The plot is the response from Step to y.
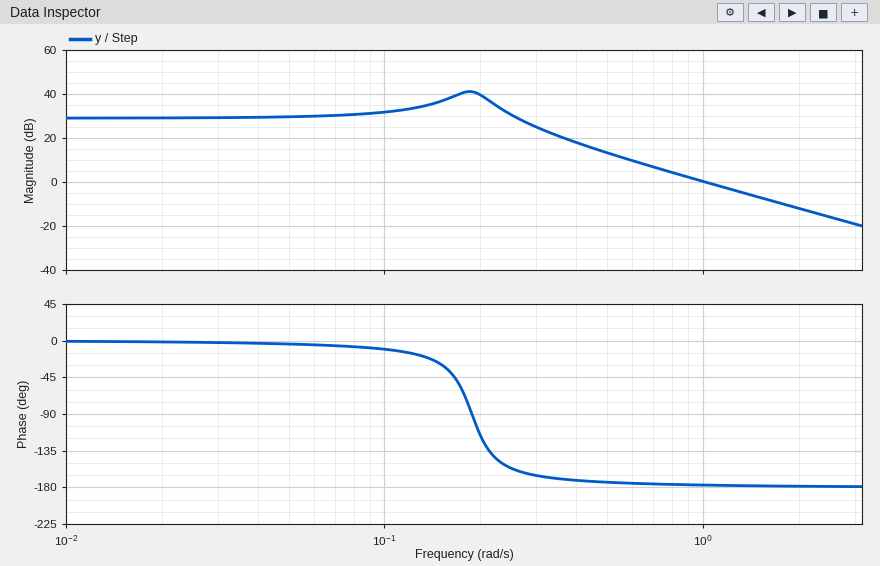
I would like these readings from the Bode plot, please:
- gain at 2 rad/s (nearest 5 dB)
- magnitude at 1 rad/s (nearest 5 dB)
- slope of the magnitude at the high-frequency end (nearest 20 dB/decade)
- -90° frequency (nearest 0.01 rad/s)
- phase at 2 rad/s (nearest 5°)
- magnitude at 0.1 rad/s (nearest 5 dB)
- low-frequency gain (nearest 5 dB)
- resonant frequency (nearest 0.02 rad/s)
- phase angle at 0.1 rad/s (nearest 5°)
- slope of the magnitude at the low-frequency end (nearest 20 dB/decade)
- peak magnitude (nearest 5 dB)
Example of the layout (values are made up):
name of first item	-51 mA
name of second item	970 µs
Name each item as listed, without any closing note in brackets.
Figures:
gain at 2 rad/s	-10 dB
magnitude at 1 rad/s	0 dB
slope of the magnitude at the high-frequency end	-40 dB/decade
-90° frequency	0.19 rad/s
phase at 2 rad/s	-180°
magnitude at 0.1 rad/s	30 dB
low-frequency gain	30 dB
resonant frequency	0.18 rad/s
phase angle at 0.1 rad/s	-10°
slope of the magnitude at the low-frequency end	0 dB/decade
peak magnitude	40 dB
